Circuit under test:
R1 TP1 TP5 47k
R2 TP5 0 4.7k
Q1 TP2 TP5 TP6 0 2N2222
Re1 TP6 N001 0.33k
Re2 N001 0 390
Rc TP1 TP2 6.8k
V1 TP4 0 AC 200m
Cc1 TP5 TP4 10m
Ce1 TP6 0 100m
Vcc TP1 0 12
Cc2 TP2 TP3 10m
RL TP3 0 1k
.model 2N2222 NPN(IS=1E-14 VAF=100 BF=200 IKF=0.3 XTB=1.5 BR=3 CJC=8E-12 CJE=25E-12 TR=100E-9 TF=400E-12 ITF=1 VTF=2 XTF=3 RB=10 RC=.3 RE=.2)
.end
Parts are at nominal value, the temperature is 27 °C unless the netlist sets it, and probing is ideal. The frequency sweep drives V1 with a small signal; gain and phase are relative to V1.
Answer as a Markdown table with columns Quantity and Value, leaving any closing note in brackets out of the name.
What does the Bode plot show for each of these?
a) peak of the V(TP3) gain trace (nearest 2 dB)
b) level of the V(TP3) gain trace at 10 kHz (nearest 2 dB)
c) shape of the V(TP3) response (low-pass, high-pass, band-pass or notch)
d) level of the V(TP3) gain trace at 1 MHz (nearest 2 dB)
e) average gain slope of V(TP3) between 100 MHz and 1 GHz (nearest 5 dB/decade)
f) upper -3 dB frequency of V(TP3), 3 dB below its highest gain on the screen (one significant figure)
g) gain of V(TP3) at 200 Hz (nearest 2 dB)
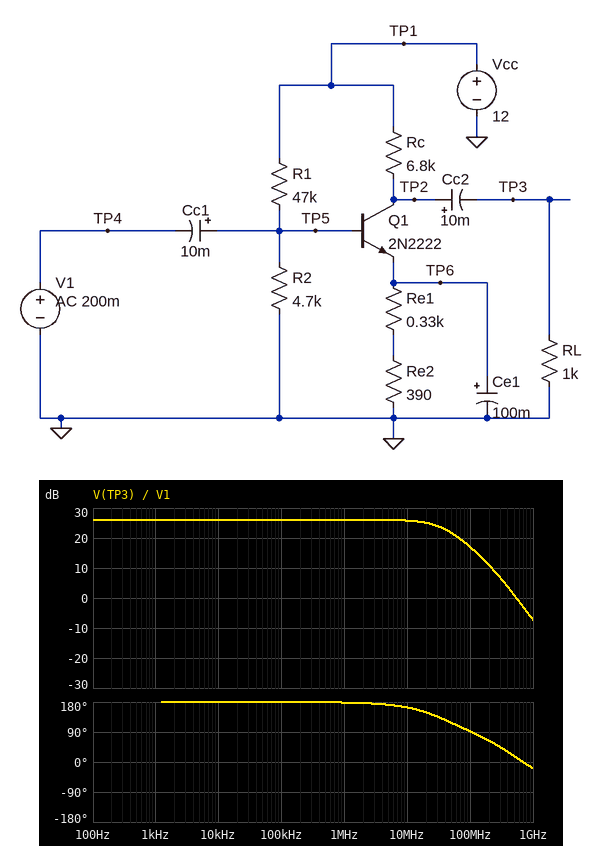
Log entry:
| Quantity | Value |
|---|---|
| peak of the V(TP3) gain trace | 26 dB |
| level of the V(TP3) gain trace at 10 kHz | 26 dB |
| shape of the V(TP3) response | low-pass |
| level of the V(TP3) gain trace at 1 MHz | 26 dB |
| average gain slope of V(TP3) between 100 MHz and 1 GHz | -25 dB/decade |
| upper -3 dB frequency of V(TP3), 3 dB below its highest gain on the screen | 40 MHz |
| gain of V(TP3) at 200 Hz | 26 dB |
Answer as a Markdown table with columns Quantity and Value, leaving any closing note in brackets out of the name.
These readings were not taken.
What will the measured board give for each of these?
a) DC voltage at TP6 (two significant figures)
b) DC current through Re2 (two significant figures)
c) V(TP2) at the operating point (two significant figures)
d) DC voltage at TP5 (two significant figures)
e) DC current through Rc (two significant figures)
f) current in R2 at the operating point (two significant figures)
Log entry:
| Quantity | Value |
|---|---|
| DC voltage at TP6 | 440 mV |
| DC current through Re2 | 610 µA |
| V(TP2) at the operating point | 7.9 V |
| DC voltage at TP5 | 1.1 V |
| DC current through Rc | 610 µA |
| current in R2 at the operating point | 230 µA |
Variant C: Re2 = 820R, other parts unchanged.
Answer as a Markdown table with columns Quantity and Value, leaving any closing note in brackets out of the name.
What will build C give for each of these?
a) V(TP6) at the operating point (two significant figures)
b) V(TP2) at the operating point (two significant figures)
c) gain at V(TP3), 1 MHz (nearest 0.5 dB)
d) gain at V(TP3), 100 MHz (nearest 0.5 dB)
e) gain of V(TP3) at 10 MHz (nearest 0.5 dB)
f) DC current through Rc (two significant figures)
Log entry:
| Quantity | Value |
|---|---|
| V(TP6) at the operating point | 450 mV |
| V(TP2) at the operating point | 9.3 V |
| gain at V(TP3), 1 MHz | 22.5 dB |
| gain at V(TP3), 100 MHz | 14.5 dB |
| gain of V(TP3) at 10 MHz | 22.0 dB |
| DC current through Rc | 390 µA |
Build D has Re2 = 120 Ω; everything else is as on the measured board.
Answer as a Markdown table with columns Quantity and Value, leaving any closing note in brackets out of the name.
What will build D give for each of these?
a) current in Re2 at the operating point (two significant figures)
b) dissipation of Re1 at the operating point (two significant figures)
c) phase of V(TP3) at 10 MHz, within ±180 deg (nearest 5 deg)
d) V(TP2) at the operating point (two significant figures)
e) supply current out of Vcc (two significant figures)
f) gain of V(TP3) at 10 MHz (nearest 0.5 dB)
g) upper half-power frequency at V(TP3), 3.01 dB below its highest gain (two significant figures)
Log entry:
| Quantity | Value |
|---|---|
| current in Re2 at the operating point | 930 µA |
| dissipation of Re1 at the operating point | 290 µW |
| phase of V(TP3) at 10 MHz, within ±180 deg | 160 deg |
| V(TP2) at the operating point | 5.7 V |
| supply current out of Vcc | 1.2 mA |
| gain of V(TP3) at 10 MHz | 29.5 dB |
| upper half-power frequency at V(TP3), 3.01 dB below its highest gain | 31 MHz |
